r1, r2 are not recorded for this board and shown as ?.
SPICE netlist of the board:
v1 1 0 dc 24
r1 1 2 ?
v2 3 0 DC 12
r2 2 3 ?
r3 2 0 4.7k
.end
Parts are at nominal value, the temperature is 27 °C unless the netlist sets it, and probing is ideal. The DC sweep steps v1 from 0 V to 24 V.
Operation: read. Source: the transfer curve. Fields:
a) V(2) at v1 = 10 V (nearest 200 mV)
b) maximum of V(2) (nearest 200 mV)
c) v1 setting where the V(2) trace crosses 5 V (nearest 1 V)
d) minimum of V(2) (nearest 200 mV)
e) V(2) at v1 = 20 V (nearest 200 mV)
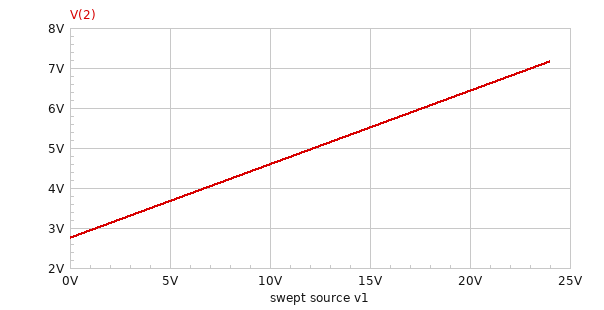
4.6 V
7.2 V
12 V
2.8 V
6.4 V
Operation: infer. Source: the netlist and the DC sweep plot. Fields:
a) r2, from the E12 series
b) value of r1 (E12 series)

12 kΩ
15 kΩ
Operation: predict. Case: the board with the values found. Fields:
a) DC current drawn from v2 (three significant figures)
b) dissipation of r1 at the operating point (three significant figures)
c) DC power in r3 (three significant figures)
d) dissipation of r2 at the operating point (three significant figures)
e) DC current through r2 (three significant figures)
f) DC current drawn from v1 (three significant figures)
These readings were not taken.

403 µA
18.9 mW
10.9 mW
1.95 mW
403 µA
1.12 mA
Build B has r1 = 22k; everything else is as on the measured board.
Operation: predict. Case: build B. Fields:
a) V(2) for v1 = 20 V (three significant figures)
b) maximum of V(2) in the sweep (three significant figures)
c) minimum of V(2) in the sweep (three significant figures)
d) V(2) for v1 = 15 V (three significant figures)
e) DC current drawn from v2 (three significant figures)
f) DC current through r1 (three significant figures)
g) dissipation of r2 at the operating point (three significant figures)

5.59 V
6.12 V
2.93 V
4.92 V
490 µA
813 µA
2.88 mW
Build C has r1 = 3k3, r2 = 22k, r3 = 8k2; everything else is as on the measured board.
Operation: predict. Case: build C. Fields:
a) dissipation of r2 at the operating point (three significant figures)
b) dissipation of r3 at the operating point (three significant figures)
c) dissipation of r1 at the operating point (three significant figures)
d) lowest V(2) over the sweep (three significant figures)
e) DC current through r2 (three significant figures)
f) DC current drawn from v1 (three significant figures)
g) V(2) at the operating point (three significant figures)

970 µW
33.7 mW
16.5 mW
1.16 V
210 µA
2.24 mA
16.6 V
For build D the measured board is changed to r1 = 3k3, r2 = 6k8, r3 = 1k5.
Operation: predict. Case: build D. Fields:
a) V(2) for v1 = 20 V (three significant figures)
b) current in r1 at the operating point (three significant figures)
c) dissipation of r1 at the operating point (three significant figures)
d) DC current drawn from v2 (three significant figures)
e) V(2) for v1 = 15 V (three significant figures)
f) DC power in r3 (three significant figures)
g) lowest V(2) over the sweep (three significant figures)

7.01 V
4.82 mA
76.7 mW
575 µA
5.65 V
43.7 mW
1.58 V
